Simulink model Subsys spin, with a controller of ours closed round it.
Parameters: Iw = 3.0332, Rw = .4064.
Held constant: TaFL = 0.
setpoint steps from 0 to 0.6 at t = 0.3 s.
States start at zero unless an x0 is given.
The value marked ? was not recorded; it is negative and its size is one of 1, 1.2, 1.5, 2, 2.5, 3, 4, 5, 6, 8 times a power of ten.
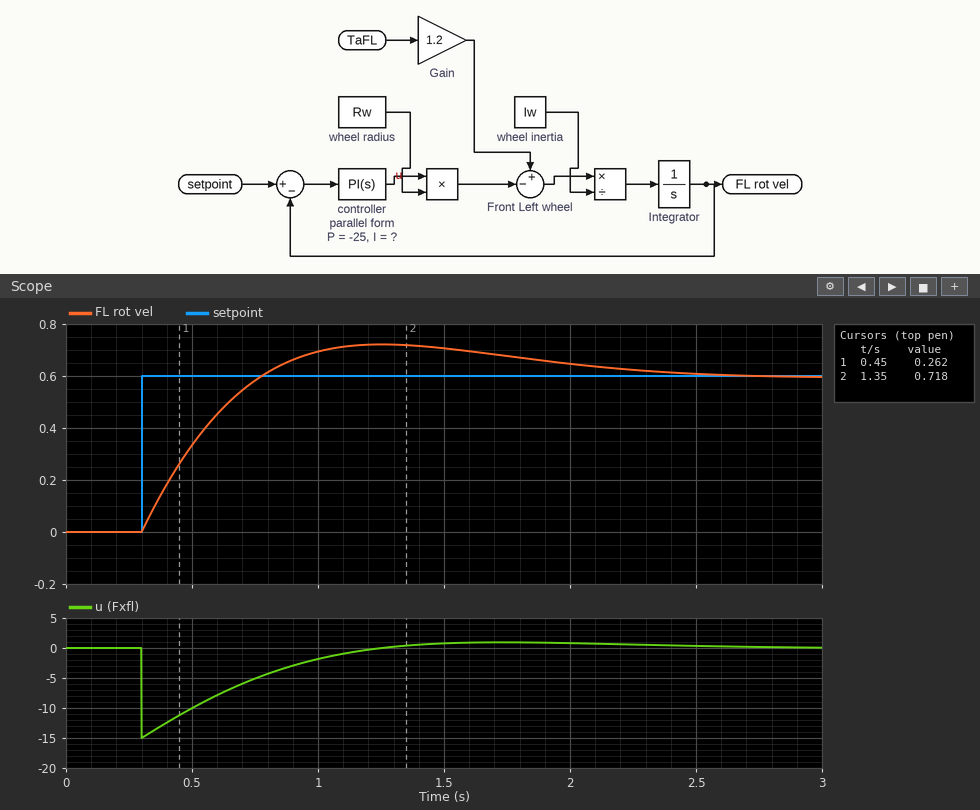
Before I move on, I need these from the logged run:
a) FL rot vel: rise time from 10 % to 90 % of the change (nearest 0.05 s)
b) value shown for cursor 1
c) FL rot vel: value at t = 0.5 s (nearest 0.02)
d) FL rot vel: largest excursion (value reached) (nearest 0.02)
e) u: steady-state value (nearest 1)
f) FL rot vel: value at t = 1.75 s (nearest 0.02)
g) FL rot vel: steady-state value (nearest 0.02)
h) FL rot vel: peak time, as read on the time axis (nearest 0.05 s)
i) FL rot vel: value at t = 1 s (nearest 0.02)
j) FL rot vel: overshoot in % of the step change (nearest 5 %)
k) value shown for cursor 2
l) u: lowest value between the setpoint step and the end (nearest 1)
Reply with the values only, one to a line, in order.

0.35 s
0.262
0.34
0.72
0
0.68
0.60
1.25 s
0.70
20 %
0.718
-15
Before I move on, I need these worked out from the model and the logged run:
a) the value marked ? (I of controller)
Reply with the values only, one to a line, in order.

-40
